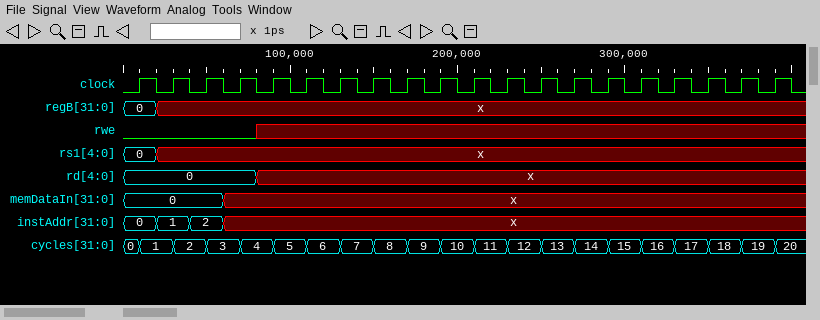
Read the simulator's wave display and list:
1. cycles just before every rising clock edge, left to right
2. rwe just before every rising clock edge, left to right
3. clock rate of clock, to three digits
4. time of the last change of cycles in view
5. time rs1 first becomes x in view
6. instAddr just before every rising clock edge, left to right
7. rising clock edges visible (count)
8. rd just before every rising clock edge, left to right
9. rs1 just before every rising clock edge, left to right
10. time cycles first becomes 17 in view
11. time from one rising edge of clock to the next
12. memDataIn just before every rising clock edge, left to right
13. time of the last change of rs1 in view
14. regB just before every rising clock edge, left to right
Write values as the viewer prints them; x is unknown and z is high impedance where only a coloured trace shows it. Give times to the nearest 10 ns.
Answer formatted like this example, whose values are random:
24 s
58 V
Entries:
0, 1, 2, 3, 4, 5, 6, 7, 8, 9, 10, 11, 12, 13, 14, 15, 16, 17, 18, 19
0 0 0 0 x x x x x x x x x x x x x x x x
50.0 MHz
390 ns
20 ns
0, 1, 2, x, x, x, x, x, x, x, x, x, x, x, x, x, x, x, x, x
20
0, 0, 0, 0, x, x, x, x, x, x, x, x, x, x, x, x, x, x, x, x
0, x, x, x, x, x, x, x, x, x, x, x, x, x, x, x, x, x, x, x
330 ns
20 ns
0, 0, 0, x, x, x, x, x, x, x, x, x, x, x, x, x, x, x, x, x
20 ns
0, x, x, x, x, x, x, x, x, x, x, x, x, x, x, x, x, x, x, x
